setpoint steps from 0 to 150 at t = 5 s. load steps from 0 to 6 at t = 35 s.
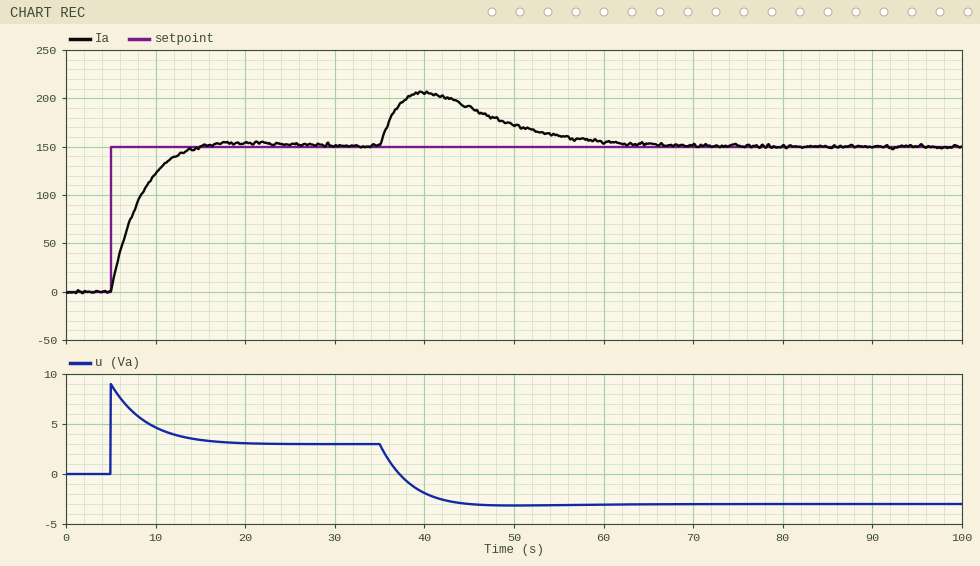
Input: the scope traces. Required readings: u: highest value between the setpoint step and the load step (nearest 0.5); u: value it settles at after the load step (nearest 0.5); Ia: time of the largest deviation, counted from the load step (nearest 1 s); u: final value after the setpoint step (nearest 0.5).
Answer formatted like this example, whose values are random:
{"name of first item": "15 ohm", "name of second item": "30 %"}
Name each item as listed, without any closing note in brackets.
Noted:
{"u: highest value between the setpoint step and the load step": "9.0", "u: value it settles at after the load step": "-3.0", "Ia: time of the largest deviation, counted from the load step": "5 s", "u: final value after the setpoint step": "3.0"}
